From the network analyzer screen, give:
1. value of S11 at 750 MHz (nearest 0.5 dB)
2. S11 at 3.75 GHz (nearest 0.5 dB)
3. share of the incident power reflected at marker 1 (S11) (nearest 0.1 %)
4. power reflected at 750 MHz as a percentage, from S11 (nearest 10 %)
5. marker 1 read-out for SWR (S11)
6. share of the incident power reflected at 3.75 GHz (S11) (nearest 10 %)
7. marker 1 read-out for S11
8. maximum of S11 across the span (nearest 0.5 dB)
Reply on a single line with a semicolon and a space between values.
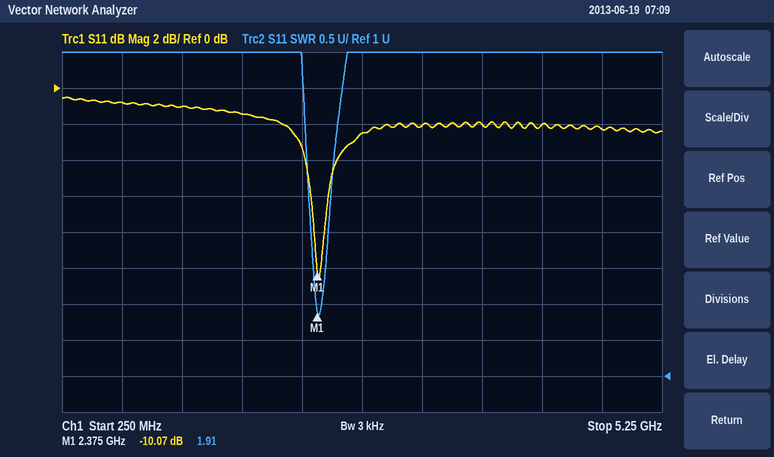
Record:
-1.0 dB; -2.0 dB; 9.8 %; 80 %; 1.91; 60 %; -10.07 dB; -0.5 dB
